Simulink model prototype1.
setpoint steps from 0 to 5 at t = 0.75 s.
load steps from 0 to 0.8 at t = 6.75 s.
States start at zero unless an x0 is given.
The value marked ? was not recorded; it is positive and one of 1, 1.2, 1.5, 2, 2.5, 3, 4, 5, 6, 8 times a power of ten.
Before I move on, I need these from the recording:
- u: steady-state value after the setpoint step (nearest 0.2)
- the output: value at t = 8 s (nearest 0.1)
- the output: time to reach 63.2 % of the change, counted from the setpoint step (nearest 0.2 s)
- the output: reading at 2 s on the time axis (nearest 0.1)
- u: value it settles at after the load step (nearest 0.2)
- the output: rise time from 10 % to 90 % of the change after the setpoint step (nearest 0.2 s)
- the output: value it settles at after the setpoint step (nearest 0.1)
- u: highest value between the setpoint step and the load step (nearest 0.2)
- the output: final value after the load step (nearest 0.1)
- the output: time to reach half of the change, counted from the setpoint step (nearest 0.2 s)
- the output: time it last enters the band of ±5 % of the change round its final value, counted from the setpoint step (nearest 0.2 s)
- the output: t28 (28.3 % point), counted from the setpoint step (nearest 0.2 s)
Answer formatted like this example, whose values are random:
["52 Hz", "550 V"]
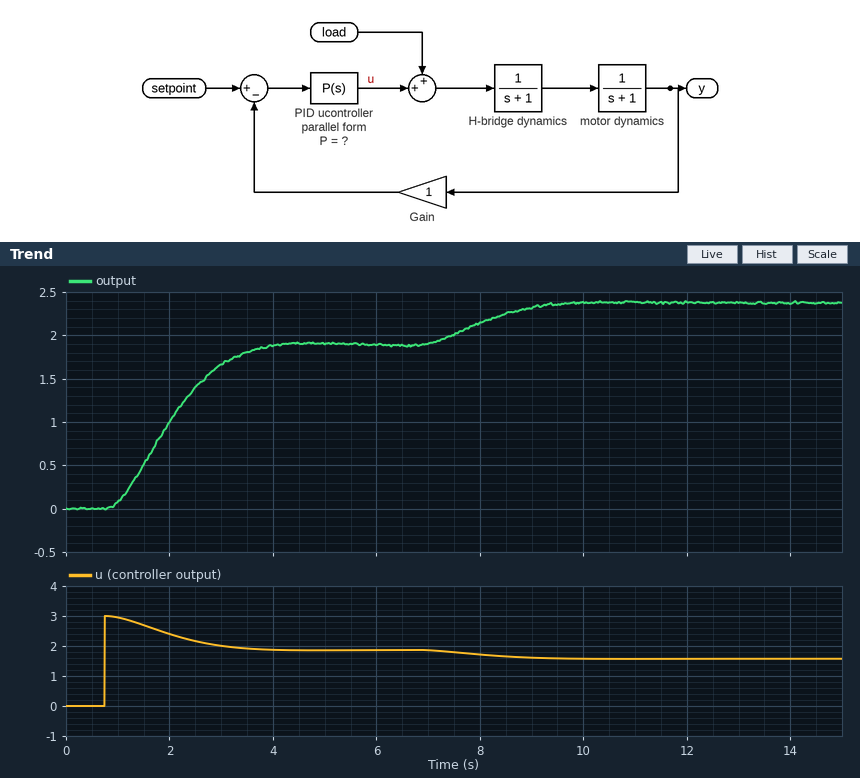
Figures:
["1.8", "2.1", "1.4 s", "1.0", "1.6", "2.0 s", "1.9", "3.0", "2.4", "1.2 s", "2.6 s", "0.8 s"]
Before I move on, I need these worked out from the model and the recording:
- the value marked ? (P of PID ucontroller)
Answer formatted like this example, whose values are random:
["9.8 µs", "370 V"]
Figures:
["0.6"]
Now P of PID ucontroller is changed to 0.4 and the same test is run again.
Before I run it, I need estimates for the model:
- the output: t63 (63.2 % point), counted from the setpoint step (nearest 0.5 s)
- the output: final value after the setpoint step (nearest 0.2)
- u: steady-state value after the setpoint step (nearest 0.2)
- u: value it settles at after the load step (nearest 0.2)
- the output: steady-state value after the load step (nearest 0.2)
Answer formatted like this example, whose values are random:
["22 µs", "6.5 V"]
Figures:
["1.5 s", "1.4", "1.4", "1.2", "2.0"]
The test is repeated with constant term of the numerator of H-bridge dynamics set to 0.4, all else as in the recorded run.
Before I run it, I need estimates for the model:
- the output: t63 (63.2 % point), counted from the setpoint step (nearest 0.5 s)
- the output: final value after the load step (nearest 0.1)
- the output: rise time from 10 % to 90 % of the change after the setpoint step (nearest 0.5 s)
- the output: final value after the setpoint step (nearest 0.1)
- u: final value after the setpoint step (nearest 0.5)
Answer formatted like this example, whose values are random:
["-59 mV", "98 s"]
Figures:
["2.0 s", "1.2", "2.5 s", "1.0", "2.5"]
